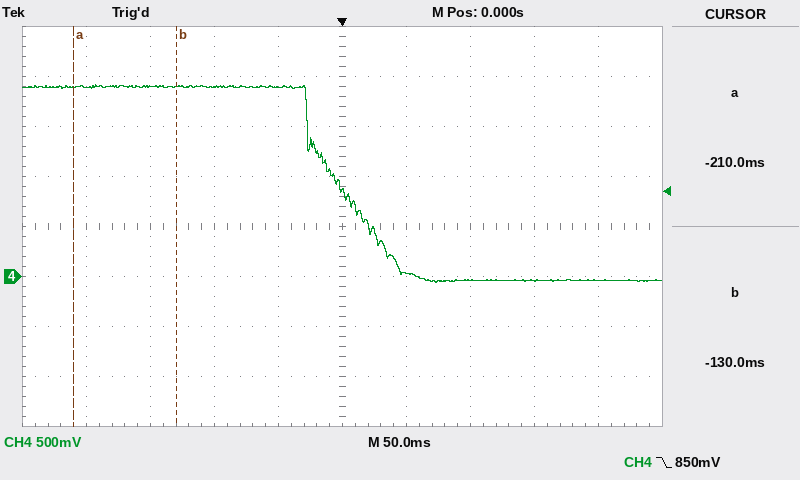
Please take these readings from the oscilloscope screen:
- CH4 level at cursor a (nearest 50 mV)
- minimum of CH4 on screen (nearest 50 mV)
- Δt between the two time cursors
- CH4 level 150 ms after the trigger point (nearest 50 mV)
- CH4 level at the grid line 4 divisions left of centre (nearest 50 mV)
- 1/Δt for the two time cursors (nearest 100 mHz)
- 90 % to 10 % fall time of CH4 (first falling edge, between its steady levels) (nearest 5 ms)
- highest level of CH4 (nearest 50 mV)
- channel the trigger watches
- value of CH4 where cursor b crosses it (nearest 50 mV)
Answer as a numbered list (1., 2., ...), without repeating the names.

1. 1.90 V
2. -50 mV
3. 80 ms
4. -50 mV
5. 1.90 V
6. 12.5 Hz
7. 70 ms
8. 1.90 V
9. CH4
10. 1.90 V
